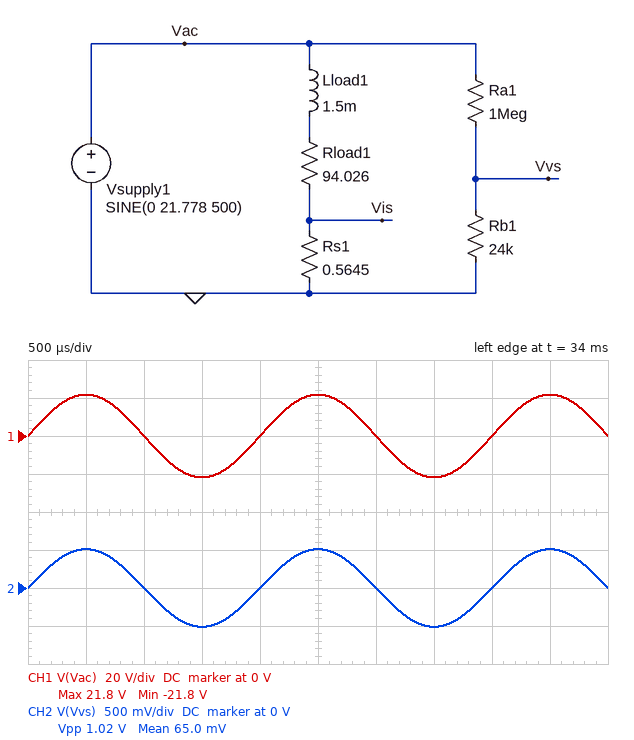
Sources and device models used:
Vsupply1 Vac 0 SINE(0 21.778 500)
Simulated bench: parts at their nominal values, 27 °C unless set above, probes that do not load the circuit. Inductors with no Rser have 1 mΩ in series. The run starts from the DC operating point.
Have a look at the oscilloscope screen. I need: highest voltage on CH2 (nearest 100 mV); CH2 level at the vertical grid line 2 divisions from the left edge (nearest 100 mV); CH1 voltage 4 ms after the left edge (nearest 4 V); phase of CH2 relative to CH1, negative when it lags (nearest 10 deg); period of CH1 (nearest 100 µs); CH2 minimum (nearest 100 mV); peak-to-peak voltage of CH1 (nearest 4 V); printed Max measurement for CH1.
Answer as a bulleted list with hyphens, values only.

- 500 mV
- 0 V
- 0 V
- 0 deg
- 2.0 ms
- -500 mV
- 44 V
- 21.8 V
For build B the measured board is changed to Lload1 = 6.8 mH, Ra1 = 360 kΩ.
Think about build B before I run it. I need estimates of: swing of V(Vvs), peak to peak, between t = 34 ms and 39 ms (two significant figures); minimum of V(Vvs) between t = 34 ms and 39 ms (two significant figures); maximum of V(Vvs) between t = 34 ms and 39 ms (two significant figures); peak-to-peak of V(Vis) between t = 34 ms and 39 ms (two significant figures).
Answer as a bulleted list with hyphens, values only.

- 2.7 V
- -1.4 V
- 1.4 V
- 250 mV
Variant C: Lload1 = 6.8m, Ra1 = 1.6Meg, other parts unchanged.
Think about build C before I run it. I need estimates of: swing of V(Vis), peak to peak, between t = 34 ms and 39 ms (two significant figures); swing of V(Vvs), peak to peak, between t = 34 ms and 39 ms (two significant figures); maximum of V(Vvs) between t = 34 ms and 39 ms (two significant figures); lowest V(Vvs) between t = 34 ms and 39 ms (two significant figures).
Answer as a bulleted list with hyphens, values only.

- 250 mV
- 640 mV
- 320 mV
- -320 mV
